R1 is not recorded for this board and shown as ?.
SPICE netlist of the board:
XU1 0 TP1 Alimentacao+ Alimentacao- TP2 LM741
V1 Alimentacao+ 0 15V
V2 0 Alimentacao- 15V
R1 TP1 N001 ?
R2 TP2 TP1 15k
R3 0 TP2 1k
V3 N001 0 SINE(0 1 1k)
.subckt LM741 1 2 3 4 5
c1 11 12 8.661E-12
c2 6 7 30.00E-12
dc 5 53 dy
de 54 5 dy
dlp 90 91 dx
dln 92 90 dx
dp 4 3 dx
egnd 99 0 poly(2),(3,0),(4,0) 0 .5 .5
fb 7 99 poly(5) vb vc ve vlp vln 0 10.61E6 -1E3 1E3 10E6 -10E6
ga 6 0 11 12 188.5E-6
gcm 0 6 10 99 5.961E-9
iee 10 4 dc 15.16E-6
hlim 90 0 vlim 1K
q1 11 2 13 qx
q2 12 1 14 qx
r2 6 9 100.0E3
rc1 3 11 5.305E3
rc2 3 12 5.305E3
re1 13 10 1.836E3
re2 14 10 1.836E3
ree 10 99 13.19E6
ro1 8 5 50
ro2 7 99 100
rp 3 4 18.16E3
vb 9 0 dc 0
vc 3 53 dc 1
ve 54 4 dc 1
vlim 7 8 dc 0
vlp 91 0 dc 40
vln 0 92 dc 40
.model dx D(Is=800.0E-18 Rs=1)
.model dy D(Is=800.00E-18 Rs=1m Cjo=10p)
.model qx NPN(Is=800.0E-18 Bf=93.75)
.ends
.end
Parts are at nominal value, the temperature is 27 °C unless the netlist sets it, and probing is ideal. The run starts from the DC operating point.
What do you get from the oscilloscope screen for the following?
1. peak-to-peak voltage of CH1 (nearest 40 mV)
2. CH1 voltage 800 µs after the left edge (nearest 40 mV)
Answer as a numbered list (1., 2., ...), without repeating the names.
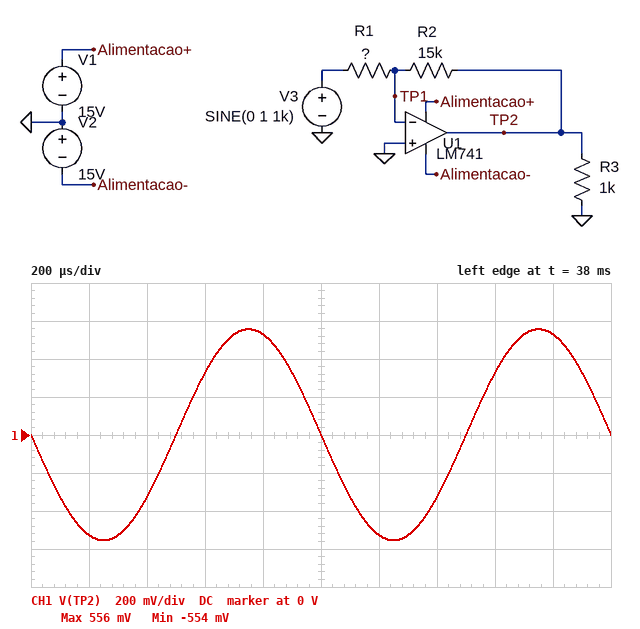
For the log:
1. 1.12 V
2. 520 mV
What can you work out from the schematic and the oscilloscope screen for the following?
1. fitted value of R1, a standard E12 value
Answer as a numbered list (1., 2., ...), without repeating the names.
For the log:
1. 27 kΩ
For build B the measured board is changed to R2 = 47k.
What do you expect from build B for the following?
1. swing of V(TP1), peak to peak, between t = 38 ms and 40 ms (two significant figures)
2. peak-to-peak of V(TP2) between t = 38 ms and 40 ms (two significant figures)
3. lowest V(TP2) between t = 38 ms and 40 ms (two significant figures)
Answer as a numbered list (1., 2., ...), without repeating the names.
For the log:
1. 3.7 mV
2. 3.5 V
3. -1.7 V
